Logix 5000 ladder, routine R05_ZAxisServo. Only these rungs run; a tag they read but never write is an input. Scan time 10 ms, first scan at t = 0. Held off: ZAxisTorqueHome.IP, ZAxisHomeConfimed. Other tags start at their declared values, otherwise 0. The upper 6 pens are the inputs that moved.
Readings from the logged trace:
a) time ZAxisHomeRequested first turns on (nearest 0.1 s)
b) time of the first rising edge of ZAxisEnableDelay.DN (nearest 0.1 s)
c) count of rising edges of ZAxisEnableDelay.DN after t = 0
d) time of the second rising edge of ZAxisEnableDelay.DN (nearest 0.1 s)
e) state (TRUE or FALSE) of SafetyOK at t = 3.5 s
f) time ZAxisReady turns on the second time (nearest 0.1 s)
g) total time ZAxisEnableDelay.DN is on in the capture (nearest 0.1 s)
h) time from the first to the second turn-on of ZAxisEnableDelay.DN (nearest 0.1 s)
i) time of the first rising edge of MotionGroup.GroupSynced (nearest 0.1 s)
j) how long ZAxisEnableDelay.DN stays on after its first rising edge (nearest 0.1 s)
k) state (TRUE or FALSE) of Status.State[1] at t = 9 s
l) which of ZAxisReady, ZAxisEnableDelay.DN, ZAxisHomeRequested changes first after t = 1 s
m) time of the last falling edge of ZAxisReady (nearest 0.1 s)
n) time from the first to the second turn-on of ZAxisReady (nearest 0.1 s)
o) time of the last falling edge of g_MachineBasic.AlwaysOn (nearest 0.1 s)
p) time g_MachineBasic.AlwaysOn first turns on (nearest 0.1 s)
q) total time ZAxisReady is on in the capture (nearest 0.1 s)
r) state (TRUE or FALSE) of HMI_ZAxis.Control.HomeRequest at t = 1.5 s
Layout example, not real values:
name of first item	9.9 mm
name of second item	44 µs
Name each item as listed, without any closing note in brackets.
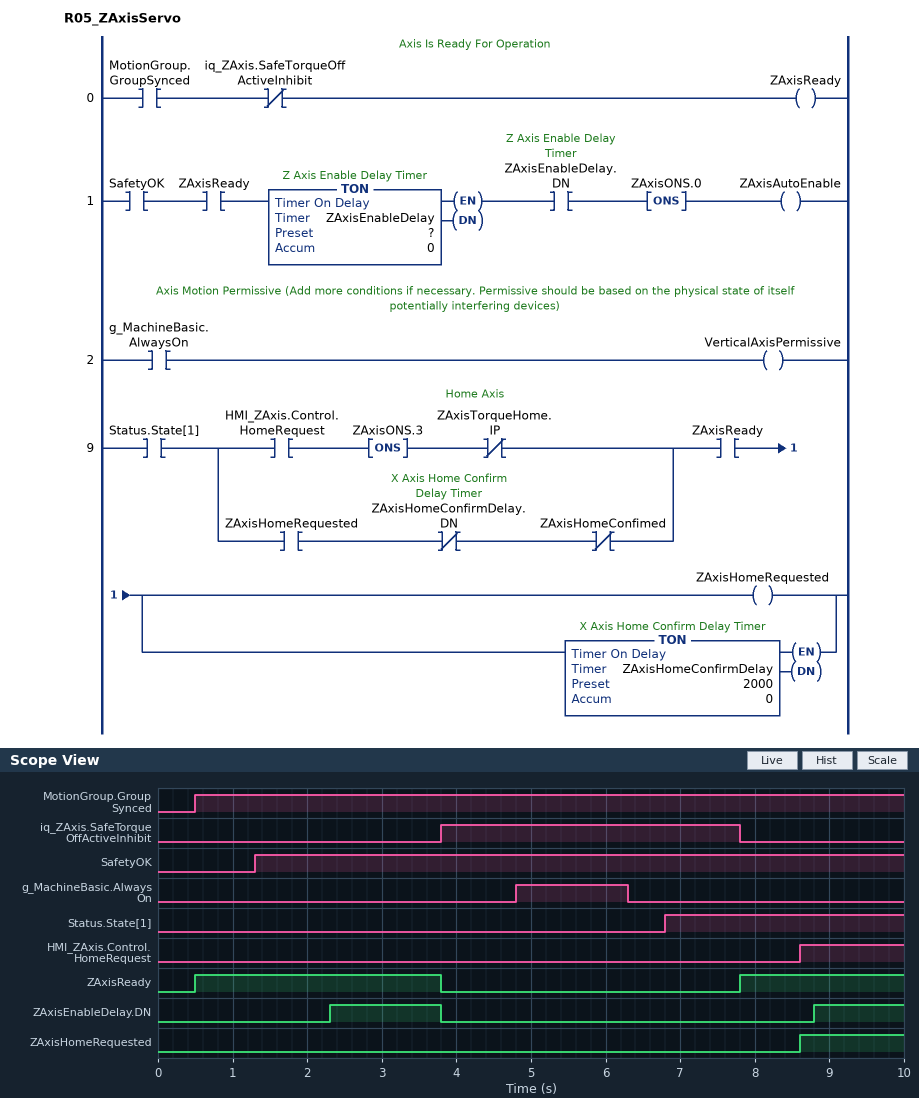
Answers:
time ZAxisHomeRequested first turns on	8.6 s
time of the first rising edge of ZAxisEnableDelay.DN	2.3 s
count of rising edges of ZAxisEnableDelay.DN after t = 0	2
time of the second rising edge of ZAxisEnableDelay.DN	8.8 s
state (TRUE or FALSE) of SafetyOK at t = 3.5 s	TRUE
time ZAxisReady turns on the second time	7.8 s
total time ZAxisEnableDelay.DN is on in the capture	2.7 s
time from the first to the second turn-on of ZAxisEnableDelay.DN	6.5 s
time of the first rising edge of MotionGroup.GroupSynced	0.5 s
how long ZAxisEnableDelay.DN stays on after its first rising edge	1.5 s
state (TRUE or FALSE) of Status.State[1] at t = 9 s	TRUE
which of ZAxisReady, ZAxisEnableDelay.DN, ZAxisHomeRequested changes first after t = 1 s	ZAxisEnableDelay.DN
time of the last falling edge of ZAxisReady	3.8 s
time from the first to the second turn-on of ZAxisReady	7.3 s
time of the last falling edge of g_MachineBasic.AlwaysOn	6.3 s
time g_MachineBasic.AlwaysOn first turns on	4.8 s
total time ZAxisReady is on in the capture	5.5 s
state (TRUE or FALSE) of HMI_ZAxis.Control.HomeRequest at t = 1.5 s	FALSE
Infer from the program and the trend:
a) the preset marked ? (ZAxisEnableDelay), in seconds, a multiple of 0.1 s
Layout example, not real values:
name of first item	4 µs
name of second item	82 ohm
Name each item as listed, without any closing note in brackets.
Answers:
the preset marked ? (ZAxisEnableDelay), in seconds, a multiple of 0.1 s	1.0 s
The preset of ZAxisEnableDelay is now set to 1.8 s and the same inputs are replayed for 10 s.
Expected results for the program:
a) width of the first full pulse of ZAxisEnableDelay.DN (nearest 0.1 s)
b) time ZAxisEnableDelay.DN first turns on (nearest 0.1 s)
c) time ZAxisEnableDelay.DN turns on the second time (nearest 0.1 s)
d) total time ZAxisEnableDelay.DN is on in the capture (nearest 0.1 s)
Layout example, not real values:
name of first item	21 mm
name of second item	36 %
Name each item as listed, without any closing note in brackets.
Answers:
width of the first full pulse of ZAxisEnableDelay.DN	0.7 s
time ZAxisEnableDelay.DN first turns on	3.1 s
time ZAxisEnableDelay.DN turns on the second time	9.6 s
total time ZAxisEnableDelay.DN is on in the capture	1.1 s
